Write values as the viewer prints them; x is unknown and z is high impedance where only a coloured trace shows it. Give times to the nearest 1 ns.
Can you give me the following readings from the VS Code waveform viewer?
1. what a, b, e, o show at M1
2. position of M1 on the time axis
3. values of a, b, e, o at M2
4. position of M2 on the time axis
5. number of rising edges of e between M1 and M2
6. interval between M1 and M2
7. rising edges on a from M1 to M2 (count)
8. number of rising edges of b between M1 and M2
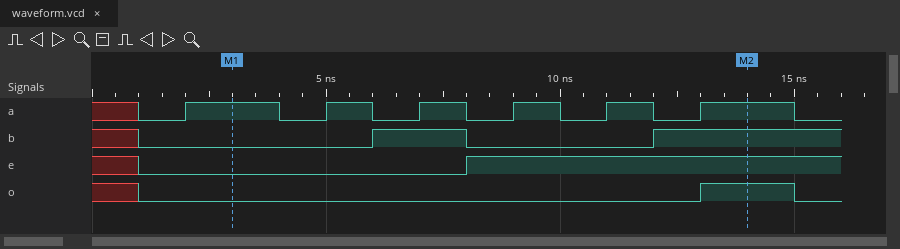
a=1, b=0, e=0, o=0
3 ns
a=1, b=1, e=1, o=1
14 ns
1
11 ns
5
2
